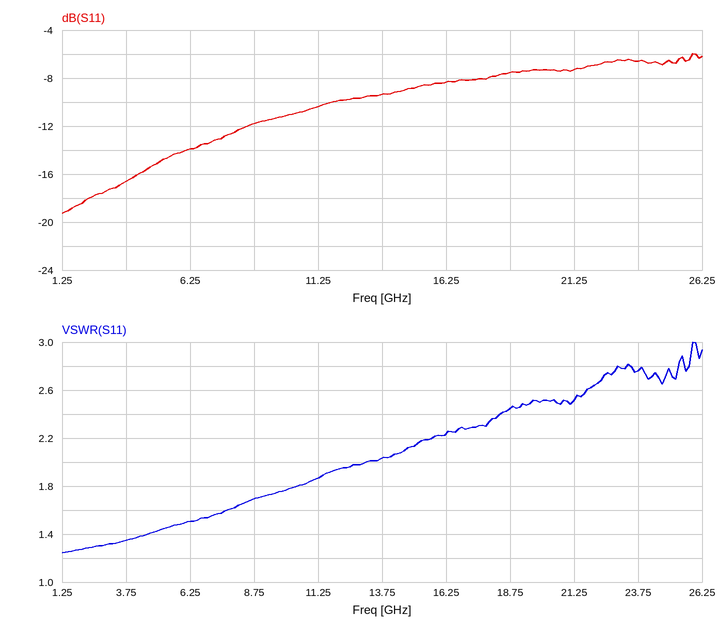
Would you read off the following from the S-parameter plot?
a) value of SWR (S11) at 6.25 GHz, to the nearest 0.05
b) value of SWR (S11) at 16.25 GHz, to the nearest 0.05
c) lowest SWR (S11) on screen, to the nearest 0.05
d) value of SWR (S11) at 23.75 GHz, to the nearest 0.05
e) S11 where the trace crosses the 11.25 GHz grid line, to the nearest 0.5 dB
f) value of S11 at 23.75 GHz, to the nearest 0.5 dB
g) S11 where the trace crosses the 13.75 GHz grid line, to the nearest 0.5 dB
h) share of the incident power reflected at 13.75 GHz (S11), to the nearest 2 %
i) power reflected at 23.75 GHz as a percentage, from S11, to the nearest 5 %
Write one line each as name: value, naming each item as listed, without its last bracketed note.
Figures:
value of SWR (S11) at 6.25 GHz, to the nearest 0.05: 1.50
value of SWR (S11) at 16.25 GHz, to the nearest 0.05: 2.25
lowest SWR (S11) on screen, to the nearest 0.05: 1.25
value of SWR (S11) at 23.75 GHz, to the nearest 0.05: 2.75
S11 where the trace crosses the 11.25 GHz grid line, to the nearest 0.5 dB: -10.5 dB
value of S11 at 23.75 GHz, to the nearest 0.5 dB: -6.5 dB
S11 where the trace crosses the 13.75 GHz grid line, to the nearest 0.5 dB: -9.5 dB
share of the incident power reflected at 13.75 GHz (S11), to the nearest 2 %: 12 %
power reflected at 23.75 GHz as a percentage, from S11, to the nearest 5 %: 20 %
